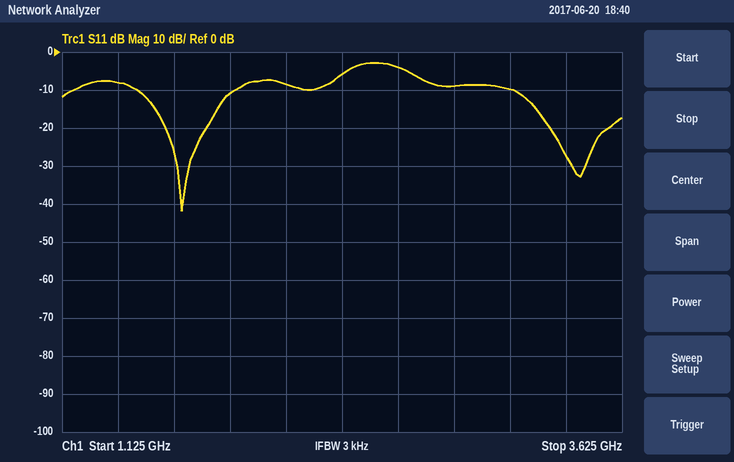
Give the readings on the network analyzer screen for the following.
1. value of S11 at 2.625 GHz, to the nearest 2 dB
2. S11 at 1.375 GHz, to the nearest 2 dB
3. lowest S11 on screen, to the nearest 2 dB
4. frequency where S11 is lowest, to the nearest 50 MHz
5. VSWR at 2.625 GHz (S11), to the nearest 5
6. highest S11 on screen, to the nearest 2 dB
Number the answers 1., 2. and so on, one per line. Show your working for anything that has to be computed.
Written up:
1. -4 dB
2. -8 dB
3. -42 dB
4. 1.65 GHz
5. |Γ| = 10^(-4/20) = 0.6310; VSWR = (1 + 0.6310)/(1 − 0.6310) ≈ 4.42, so 5 to the nearest 5
6. -2 dB
